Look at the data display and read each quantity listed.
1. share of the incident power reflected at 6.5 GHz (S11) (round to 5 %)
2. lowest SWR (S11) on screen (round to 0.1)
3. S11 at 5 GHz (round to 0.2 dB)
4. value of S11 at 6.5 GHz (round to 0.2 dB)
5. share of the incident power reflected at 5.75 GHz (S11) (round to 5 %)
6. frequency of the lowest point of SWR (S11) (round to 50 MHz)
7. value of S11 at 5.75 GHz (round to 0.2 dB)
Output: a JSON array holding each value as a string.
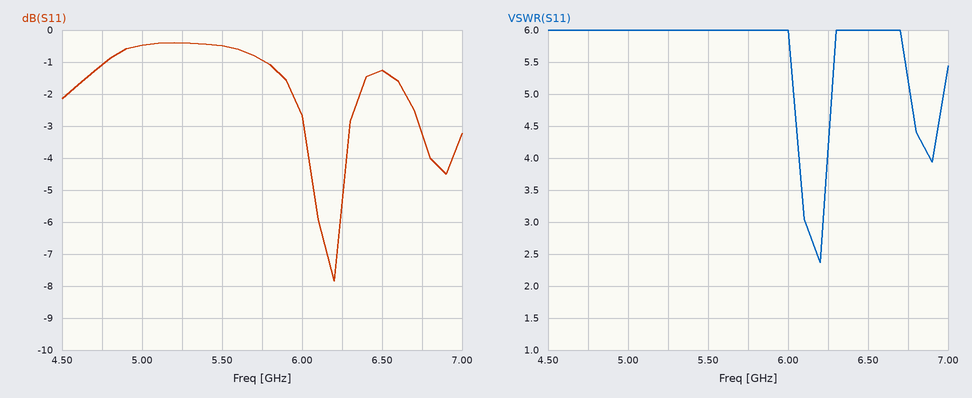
["75 %", "2.4", "-0.4 dB", "-1.2 dB", "80 %", "6.20 GHz", "-1.0 dB"]
